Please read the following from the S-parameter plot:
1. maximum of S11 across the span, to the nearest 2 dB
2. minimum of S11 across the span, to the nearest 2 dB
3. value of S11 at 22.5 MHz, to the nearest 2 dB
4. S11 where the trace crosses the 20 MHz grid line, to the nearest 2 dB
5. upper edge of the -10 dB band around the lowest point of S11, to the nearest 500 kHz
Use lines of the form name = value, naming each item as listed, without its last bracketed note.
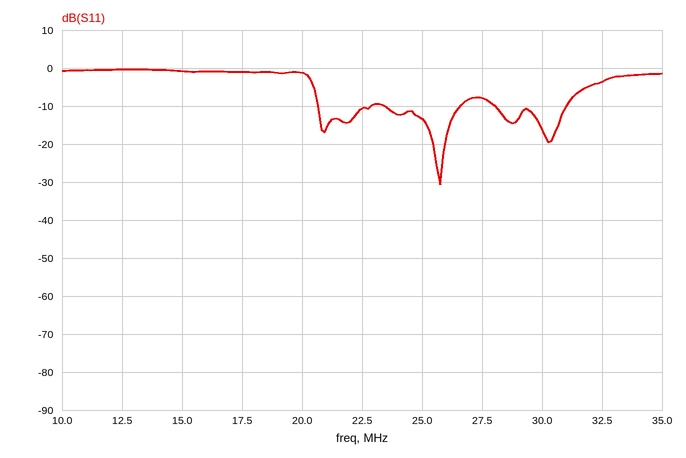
maximum of S11 across the span, to the nearest 2 dB = 0 dB
minimum of S11 across the span, to the nearest 2 dB = -30 dB
value of S11 at 22.5 MHz, to the nearest 2 dB = -10 dB
S11 where the trace crosses the 20 MHz grid line, to the nearest 2 dB = -2 dB
upper edge of the -10 dB band around the lowest point of S11, to the nearest 500 kHz = 26.5 MHz
